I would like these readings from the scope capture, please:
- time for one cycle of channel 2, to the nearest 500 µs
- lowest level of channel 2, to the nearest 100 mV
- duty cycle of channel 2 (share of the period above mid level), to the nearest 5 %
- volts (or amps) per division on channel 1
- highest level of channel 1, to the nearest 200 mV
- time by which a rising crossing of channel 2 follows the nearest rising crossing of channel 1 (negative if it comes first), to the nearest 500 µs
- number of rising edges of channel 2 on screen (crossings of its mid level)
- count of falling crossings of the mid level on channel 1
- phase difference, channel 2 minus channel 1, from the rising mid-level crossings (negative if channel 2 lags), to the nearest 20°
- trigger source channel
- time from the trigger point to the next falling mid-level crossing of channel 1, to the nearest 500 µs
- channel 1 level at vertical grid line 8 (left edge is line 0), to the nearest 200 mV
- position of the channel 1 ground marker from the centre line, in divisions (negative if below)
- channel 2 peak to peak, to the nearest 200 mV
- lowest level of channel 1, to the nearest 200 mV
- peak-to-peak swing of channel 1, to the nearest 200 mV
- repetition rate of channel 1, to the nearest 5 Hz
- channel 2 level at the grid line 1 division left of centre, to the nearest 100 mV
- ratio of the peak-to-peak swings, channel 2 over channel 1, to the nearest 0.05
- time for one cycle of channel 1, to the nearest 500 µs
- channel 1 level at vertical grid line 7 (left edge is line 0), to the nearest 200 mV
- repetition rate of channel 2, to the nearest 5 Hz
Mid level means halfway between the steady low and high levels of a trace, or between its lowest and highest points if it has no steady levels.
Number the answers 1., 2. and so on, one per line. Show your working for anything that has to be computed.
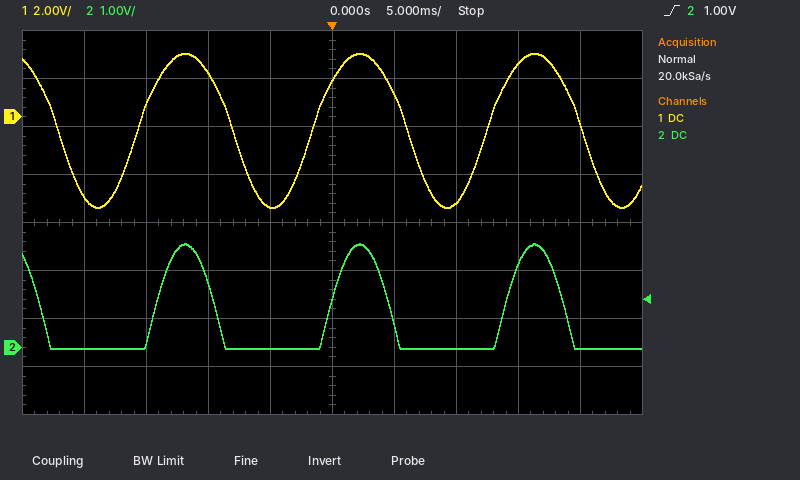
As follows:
1. 14.0 ms
2. 0.0 V
3. 30 %
4. 2 V
5. 2.6 V
6. +1.5 ms
7. 3
8. 4
9. −360° × (+1.5 ms) / 14.0 ms ≈ -38.6°, so -40° to the nearest 20°
10. channel 2
11. 6.0 ms
12. 2.2 V
13. +2.2 div
14. 2.2 V
15. -3.8 V
16. 2.6 V − (-3.8 V) = 6.4 V
17. 1 / 14.0 ms ≈ 71.4 Hz, so 70 Hz to the nearest 5 Hz
18. 0.0 V
19. 2.2 V / 6.4 V ≈ 0.344, so 0.35 to the nearest 0.05
20. 14.0 ms
21. -3.6 V
22. 1 / 14.0 ms ≈ 71.4 Hz, so 70 Hz to the nearest 5 Hz
